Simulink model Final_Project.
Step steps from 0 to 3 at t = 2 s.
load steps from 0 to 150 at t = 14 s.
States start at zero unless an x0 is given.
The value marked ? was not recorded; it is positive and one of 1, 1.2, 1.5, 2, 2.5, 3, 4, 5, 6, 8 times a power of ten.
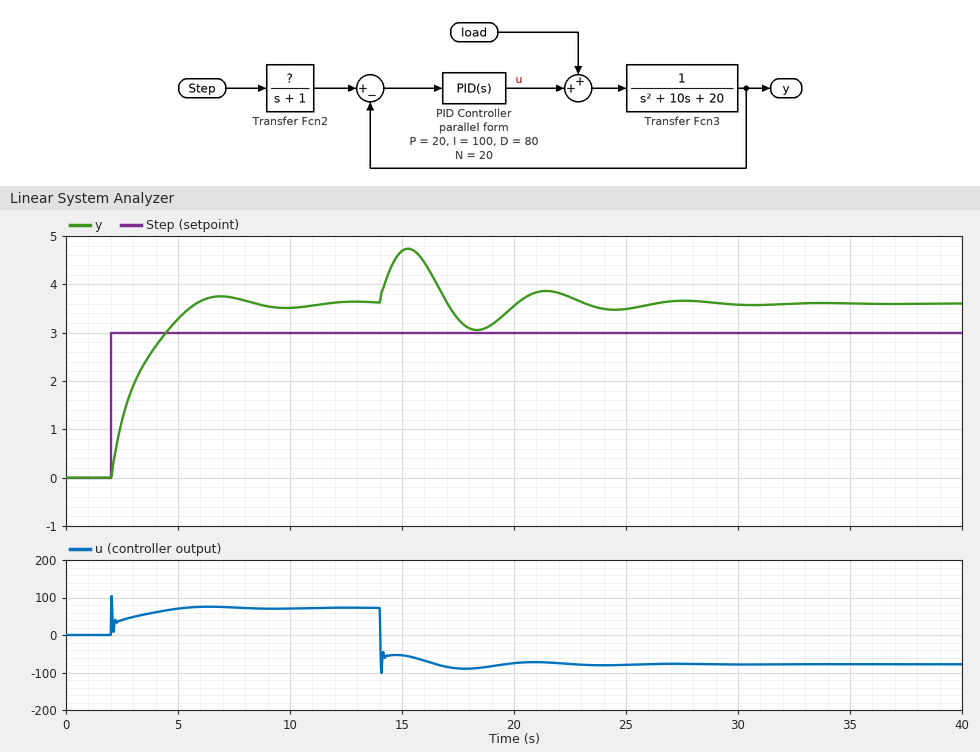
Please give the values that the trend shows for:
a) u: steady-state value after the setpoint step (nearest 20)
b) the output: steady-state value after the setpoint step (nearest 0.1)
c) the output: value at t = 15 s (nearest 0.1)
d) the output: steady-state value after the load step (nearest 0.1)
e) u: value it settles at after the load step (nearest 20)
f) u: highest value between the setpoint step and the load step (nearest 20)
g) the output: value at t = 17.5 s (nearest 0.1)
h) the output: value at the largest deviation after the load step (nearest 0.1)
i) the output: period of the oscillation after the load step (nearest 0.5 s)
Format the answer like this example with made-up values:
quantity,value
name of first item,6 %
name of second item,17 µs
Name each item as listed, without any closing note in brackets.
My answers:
quantity,value
u: steady-state value after the setpoint step,80
the output: steady-state value after the setpoint step,3.6
the output: value at t = 15 s,4.7
the output: steady-state value after the load step,3.6
u: value it settles at after the load step,-80
u: highest value between the setpoint step and the load step,100
the output: value at t = 17.5 s,3.3
the output: value at the largest deviation after the load step,4.7
the output: period of the oscillation after the load step,6.0 s
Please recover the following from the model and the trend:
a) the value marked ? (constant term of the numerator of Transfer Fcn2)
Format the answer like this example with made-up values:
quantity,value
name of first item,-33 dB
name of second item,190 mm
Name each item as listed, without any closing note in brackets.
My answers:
quantity,value
the value marked ?,1.2
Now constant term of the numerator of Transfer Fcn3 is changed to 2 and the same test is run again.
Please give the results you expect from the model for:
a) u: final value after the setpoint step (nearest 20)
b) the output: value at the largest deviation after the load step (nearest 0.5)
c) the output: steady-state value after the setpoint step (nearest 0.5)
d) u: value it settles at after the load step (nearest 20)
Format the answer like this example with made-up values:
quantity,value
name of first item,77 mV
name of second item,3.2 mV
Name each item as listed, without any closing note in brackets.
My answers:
quantity,value
u: final value after the setpoint step,40
the output: value at the largest deviation after the load step,5.0
the output: steady-state value after the setpoint step,3.5
u: value it settles at after the load step,-120
